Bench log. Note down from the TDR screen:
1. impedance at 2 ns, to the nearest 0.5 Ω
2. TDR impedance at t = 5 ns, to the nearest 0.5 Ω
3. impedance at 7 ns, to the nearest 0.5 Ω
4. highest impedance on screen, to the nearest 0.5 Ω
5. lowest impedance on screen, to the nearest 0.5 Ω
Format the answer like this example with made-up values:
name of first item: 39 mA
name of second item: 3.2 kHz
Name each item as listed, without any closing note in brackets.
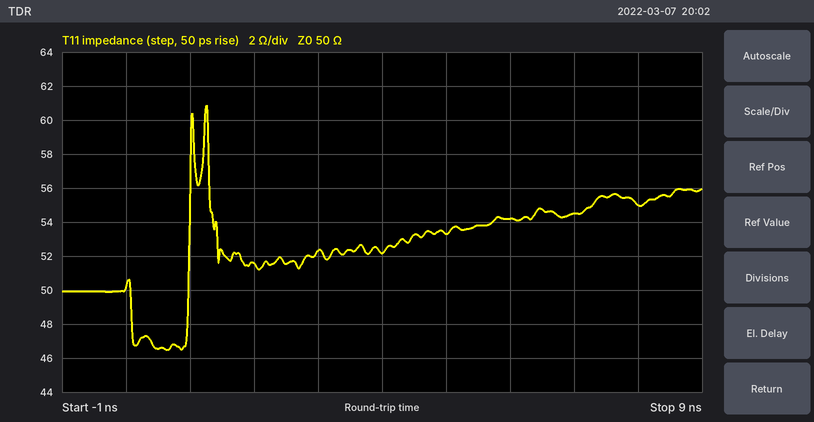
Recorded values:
impedance at 2 ns, to the nearest 0.5 Ω: 51.5 Ω
TDR impedance at t = 5 ns, to the nearest 0.5 Ω: 53.5 Ω
impedance at 7 ns, to the nearest 0.5 Ω: 54.5 Ω
highest impedance on screen, to the nearest 0.5 Ω: 61.0 Ω
lowest impedance on screen, to the nearest 0.5 Ω: 46.5 Ω
